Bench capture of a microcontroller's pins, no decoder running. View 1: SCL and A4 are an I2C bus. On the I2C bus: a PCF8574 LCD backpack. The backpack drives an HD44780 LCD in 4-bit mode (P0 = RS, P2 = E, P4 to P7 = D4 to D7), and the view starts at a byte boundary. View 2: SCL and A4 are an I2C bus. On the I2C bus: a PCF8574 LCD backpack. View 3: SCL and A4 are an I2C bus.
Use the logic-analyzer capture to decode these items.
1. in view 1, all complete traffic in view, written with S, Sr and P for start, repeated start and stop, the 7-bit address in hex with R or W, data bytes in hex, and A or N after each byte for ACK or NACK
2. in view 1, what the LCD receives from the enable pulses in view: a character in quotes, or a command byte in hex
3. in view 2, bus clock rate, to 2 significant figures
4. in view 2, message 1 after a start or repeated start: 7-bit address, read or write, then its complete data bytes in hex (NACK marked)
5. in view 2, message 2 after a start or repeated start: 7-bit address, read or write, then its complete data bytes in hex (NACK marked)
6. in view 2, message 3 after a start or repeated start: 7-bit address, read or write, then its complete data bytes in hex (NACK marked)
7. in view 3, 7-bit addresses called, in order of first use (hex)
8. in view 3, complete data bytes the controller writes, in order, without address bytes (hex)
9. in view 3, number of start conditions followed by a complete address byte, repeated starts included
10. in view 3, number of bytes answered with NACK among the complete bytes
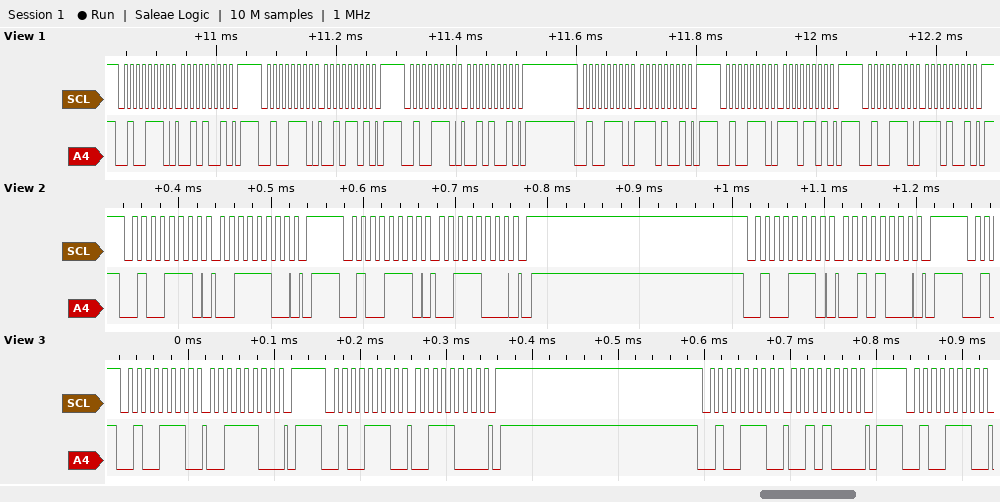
S 27W A 29 A P S 27W A 2D A P S 27W A 29 A P S 27W A E9 A P S 27W A ED A P S 27W A E9 A P
'.'
100 kHz
0x27 write: 3C
0x27 write: 38
0x27 write: 28
0x27
3C 38 28
4
0
